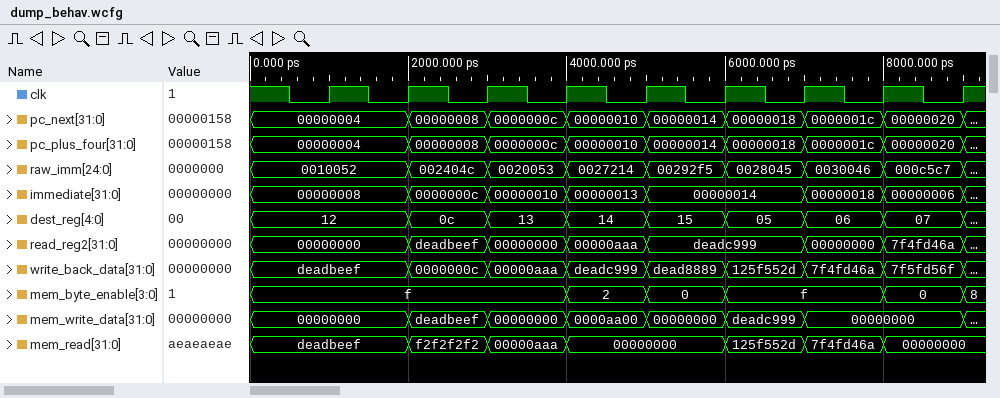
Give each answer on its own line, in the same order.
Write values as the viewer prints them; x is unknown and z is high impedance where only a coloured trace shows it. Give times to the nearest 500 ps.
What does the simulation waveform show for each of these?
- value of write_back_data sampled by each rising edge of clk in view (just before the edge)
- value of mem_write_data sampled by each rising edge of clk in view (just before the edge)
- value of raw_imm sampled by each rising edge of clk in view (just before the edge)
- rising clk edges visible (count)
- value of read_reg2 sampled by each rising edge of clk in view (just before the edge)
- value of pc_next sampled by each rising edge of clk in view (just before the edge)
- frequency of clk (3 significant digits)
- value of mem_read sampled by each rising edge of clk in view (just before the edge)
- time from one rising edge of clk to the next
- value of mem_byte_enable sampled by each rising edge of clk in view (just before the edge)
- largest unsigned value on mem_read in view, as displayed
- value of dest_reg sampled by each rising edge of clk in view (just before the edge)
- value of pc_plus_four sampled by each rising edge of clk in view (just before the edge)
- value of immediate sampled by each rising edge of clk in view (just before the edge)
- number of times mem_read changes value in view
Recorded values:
deadbeef, deadbeef, 0000000c, 00000aaa, deadc999, dead8889, 125f552d, 7f4fd46a, 7f5fd56f
00000000, 00000000, deadbeef, 00000000, 0000aa00, 00000000, deadc999, 00000000, 00000000
0010052, 0010052, 002404c, 0020053, 0027214, 00292f5, 0028045, 0030046, 000c5c7
9
00000000, 00000000, deadbeef, 00000000, 00000aaa, deadc999, deadc999, 00000000, 7f4fd46a
00000004, 00000004, 00000008, 0000000c, 00000010, 00000014, 00000018, 0000001c, 00000020
1.00 GHz
deadbeef, deadbeef, f2f2f2f2, 00000aaa, 00000000, 00000000, 125f552d, 7f4fd46a, 00000000
1000 ps
f, f, f, f, 2, 0, f, f, 0
f2f2f2f2
12, 12, 0c, 13, 14, 15, 05, 06, 07
00000004, 00000004, 00000008, 0000000c, 00000010, 00000014, 00000018, 0000001c, 00000020
00000008, 00000008, 0000000c, 00000010, 00000013, 00000014, 00000014, 00000018, 00000006
6
